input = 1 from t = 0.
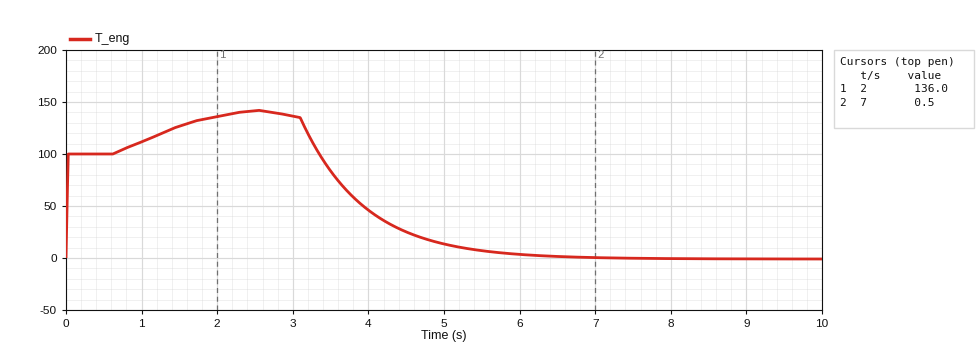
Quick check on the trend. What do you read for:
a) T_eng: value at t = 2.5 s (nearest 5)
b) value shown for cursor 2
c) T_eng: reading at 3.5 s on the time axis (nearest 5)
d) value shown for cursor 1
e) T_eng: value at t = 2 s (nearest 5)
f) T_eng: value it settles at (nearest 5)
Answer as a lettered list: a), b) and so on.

a) 140
b) 0.5
c) 85
d) 136.0
e) 135
f) 0
